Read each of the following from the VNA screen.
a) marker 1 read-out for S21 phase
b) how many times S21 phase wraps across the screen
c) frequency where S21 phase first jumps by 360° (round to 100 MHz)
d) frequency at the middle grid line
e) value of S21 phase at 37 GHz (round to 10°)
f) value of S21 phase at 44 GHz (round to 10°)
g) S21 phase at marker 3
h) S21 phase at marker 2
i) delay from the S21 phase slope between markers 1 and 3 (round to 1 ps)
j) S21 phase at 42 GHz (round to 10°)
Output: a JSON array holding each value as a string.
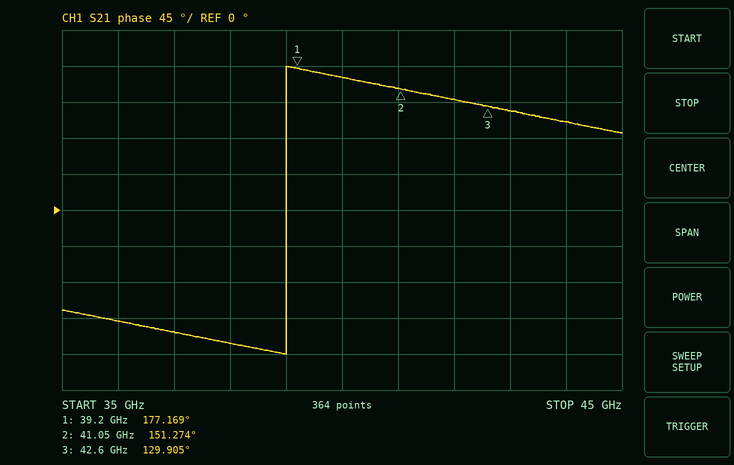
["177.169°", "1", "39.0 GHz", "40 GHz", "-150°", "110°", "129.905°", "151.274°", "39 ps", "140°"]
